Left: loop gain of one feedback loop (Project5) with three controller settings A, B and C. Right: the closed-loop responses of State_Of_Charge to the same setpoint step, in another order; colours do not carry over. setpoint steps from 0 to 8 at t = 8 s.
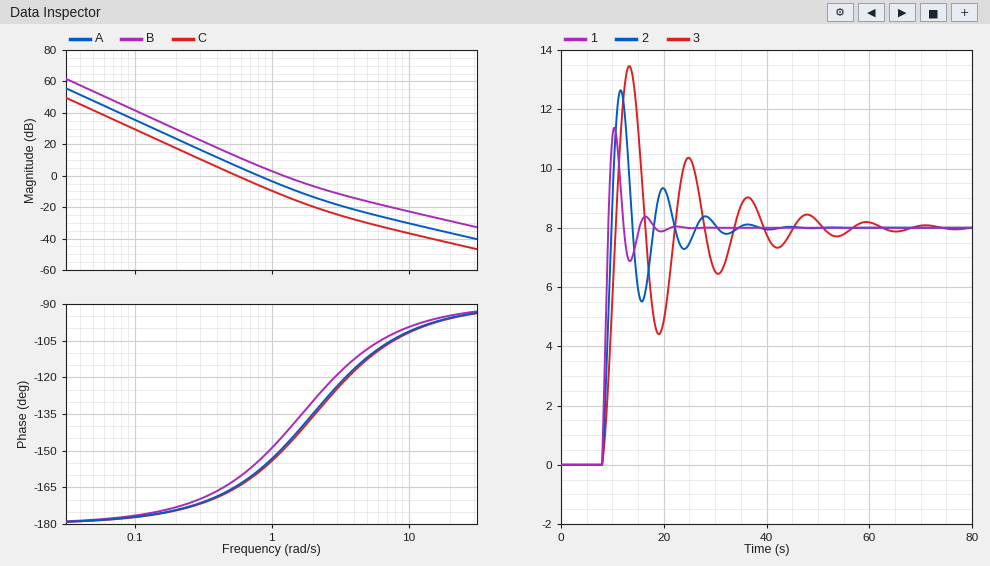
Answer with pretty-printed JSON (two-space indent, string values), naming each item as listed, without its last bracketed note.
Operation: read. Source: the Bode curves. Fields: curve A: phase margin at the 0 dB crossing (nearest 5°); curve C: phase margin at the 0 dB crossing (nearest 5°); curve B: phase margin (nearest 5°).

{
  "curve A: phase margin at the 0 dB crossing": "20°",
  "curve C: phase margin at the 0 dB crossing": "15°",
  "curve B: phase margin": "35°"
}
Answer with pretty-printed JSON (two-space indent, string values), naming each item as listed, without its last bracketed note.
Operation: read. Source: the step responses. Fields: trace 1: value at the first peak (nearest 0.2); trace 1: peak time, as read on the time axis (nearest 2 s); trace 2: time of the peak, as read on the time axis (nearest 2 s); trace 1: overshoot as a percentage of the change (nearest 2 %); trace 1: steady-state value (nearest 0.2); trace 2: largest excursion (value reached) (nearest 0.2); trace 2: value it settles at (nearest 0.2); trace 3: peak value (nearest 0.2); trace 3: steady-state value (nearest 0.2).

{
  "trace 1: value at the first peak": "11.4",
  "trace 1: peak time, as read on the time axis": "10 s",
  "trace 2: time of the peak, as read on the time axis": "12 s",
  "trace 1: overshoot as a percentage of the change": "42 %",
  "trace 1: steady-state value": "8.0",
  "trace 2: largest excursion (value reached)": "12.6",
  "trace 2: value it settles at": "8.0",
  "trace 3: peak value": "13.4",
  "trace 3: steady-state value": "8.0"
}
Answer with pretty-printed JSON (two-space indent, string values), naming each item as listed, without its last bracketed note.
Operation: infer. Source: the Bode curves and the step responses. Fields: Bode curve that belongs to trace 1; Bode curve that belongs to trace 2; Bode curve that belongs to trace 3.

{
  "Bode curve that belongs to trace 1": "B",
  "Bode curve that belongs to trace 2": "A",
  "Bode curve that belongs to trace 3": "C"
}
